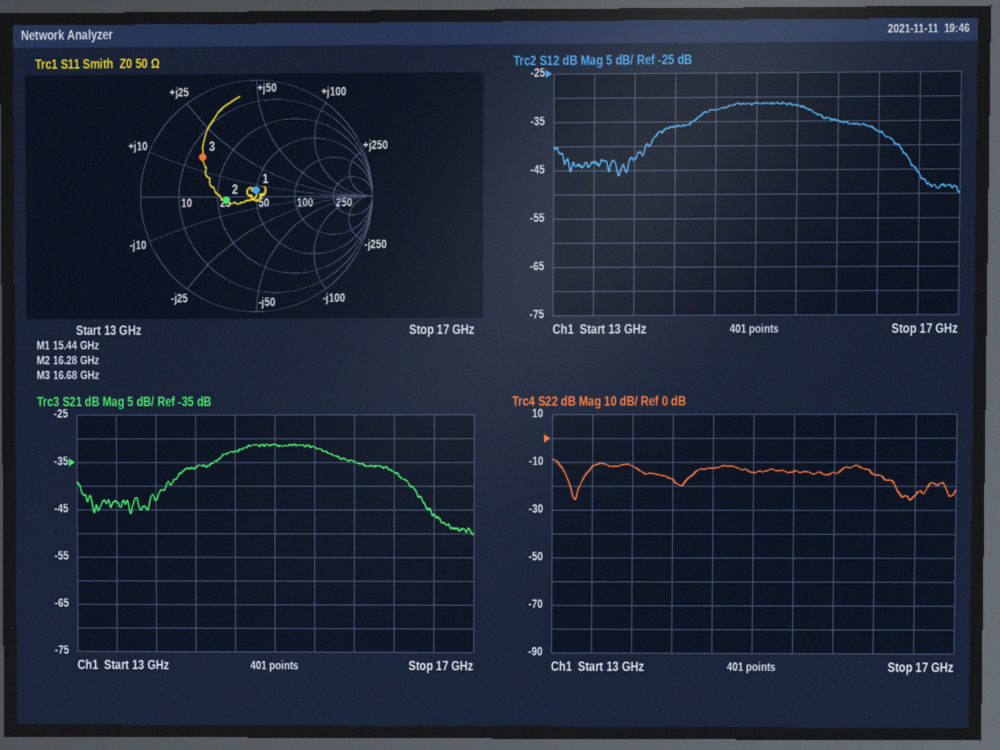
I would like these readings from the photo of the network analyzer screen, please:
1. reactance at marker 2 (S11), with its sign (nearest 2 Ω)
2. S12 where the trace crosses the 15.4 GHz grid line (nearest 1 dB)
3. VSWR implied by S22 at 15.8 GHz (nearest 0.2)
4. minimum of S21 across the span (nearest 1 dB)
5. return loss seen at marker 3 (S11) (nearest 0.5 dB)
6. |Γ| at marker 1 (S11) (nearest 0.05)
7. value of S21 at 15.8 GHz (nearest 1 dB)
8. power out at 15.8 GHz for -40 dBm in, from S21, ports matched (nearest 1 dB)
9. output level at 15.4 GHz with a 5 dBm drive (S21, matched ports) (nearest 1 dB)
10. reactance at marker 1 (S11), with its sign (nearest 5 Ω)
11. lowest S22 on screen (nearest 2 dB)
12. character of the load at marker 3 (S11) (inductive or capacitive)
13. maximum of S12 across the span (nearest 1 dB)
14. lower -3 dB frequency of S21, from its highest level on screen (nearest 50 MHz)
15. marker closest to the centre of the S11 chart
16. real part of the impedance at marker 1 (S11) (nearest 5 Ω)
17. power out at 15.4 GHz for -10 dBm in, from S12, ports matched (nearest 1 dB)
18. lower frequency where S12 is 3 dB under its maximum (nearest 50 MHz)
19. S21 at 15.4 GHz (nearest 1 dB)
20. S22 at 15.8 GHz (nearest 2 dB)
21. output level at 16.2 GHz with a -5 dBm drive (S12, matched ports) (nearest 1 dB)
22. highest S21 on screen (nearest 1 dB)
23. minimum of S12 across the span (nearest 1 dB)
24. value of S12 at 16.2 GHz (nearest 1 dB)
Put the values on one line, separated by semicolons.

-2 Ω; -32 dB; 1.4; -50 dB; 5.0 dB; 0.05; -35 dB; -75 dBm; -27 dBm; +5 Ω; -26 dB; inductive; -31 dB; 14.45 GHz; marker 1; 50 Ω; -42 dBm; 14.40 GHz; -32 dB; -14 dB; -42 dBm; -31 dB; -50 dB; -37 dB
